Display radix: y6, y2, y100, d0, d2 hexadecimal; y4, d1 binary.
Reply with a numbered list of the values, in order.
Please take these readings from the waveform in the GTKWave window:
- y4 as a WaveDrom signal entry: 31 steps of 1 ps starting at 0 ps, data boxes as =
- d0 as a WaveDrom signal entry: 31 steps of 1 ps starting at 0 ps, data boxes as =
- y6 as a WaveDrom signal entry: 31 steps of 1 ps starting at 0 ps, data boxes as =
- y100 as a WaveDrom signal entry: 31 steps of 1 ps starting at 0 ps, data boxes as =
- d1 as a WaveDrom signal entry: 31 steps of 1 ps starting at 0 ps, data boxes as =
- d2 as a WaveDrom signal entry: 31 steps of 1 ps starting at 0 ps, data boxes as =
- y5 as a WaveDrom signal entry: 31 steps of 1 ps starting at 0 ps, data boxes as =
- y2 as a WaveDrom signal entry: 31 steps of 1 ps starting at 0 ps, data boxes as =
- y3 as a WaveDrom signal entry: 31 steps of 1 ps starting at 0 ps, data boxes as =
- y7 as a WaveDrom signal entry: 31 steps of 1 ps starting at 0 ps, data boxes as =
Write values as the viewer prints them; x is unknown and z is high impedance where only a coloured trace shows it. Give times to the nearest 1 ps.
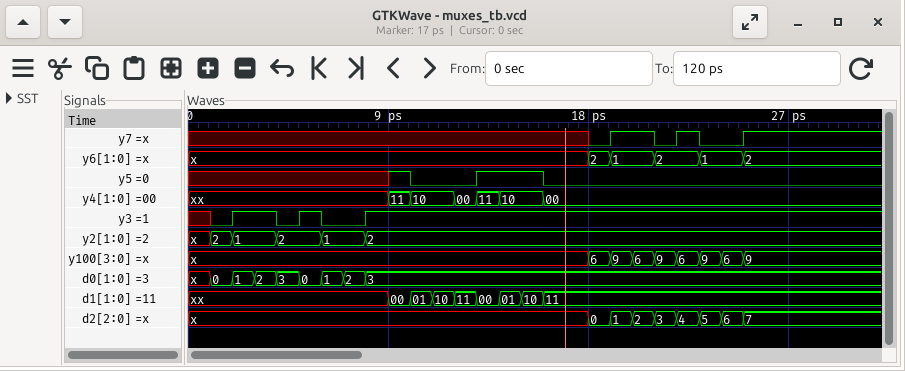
1. {name: 'y4', wave: 'x........==.===.=..............', data: '11 10 00 11 10 00'}
2. {name: 'd0', wave: 'x========......................', data: '0 1 2 3 0 1 2 3'}
3. {name: 'y6', wave: 'x.................==.=.=.=.....', data: '2 1 2 1 2'}
4. {name: 'y100', wave: 'x.................========.....', data: '6 9 6 9 6 9 6 9'}
5. {name: 'd1', wave: 'x........========..............', data: '00 01 10 11 00 01 10 11'}
6. {name: 'd2', wave: 'x.................========.....', data: '0 1 2 3 4 5 6 7'}
7. {name: 'y5', wave: 'x........10..1..0..............'}
8. {name: 'y2', wave: 'x==.=.=.=......................', data: '2 1 2 1 2'}
9. {name: 'y3', wave: 'x01.010.1......................'}
10. {name: 'y7', wave: 'x.................01.010.1.....'}
